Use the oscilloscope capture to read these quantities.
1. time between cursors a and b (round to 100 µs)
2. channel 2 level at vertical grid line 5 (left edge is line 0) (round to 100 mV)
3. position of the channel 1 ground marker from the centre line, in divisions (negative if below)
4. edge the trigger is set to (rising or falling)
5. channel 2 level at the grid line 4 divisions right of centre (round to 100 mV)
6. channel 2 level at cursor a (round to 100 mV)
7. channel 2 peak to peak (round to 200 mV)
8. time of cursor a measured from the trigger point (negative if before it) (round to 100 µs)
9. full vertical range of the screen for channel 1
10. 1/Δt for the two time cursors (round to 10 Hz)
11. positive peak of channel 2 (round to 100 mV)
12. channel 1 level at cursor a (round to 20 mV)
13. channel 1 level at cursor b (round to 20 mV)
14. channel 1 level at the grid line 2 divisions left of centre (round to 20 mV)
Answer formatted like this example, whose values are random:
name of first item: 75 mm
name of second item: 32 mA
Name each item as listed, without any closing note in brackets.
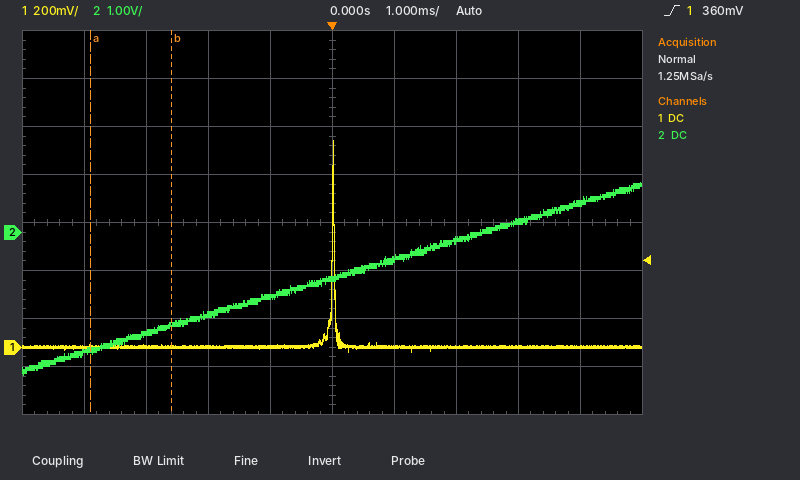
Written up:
time between cursors a and b: 1.3 ms
channel 2 level at vertical grid line 5 (left edge is line 0): -1.0 V
position of the channel 1 ground marker from the centre line, in divisions: -2.6 div
edge the trigger is set to: rising
channel 2 level at the grid line 4 divisions right of centre: 600 mV
channel 2 level at cursor a: -2.5 V
channel 2 peak to peak: 4.0 V
time of cursor a measured from the trigger point (negative if before it): -3.9 ms
full vertical range of the screen for channel 1: 1.6 V
1/Δt for the two time cursors: 770 Hz
positive peak of channel 2: 1.0 V
channel 1 level at cursor a: 0 mV
channel 1 level at cursor b: 0 mV
channel 1 level at the grid line 2 divisions left of centre: 0 mV
